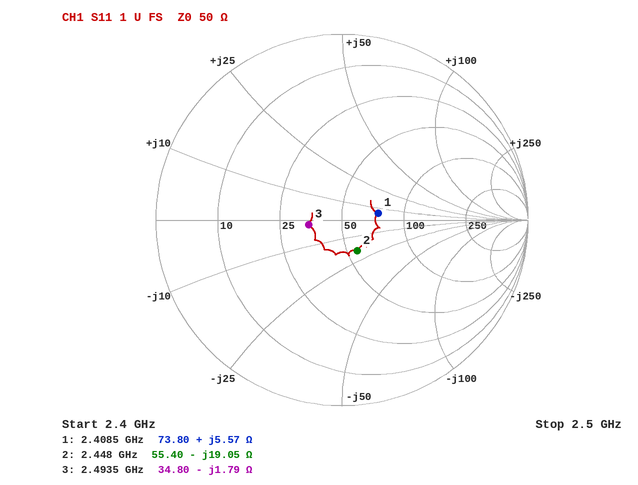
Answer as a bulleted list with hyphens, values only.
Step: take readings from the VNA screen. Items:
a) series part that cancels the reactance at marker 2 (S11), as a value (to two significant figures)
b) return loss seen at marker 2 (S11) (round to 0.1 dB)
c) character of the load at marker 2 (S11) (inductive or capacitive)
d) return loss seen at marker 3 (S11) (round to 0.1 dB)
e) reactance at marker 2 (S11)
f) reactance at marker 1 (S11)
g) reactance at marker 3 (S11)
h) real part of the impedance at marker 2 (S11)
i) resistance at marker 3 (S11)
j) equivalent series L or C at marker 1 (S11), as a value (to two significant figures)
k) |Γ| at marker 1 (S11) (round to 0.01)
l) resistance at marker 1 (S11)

- 1.2 nH
- 14.7 dB
- capacitive
- 14.9 dB
- -19.05 Ω
- +5.57 Ω
- -1.79 Ω
- 55.40 Ω
- 34.80 Ω
- 370 pH
- 0.20
- 73.80 Ω
